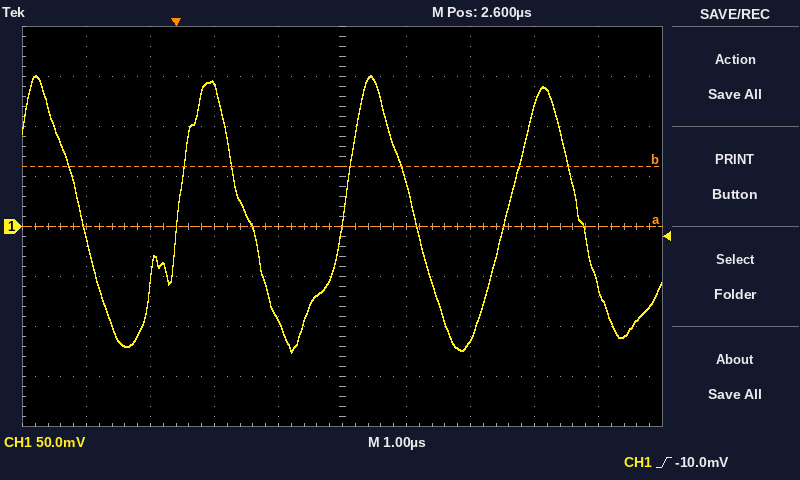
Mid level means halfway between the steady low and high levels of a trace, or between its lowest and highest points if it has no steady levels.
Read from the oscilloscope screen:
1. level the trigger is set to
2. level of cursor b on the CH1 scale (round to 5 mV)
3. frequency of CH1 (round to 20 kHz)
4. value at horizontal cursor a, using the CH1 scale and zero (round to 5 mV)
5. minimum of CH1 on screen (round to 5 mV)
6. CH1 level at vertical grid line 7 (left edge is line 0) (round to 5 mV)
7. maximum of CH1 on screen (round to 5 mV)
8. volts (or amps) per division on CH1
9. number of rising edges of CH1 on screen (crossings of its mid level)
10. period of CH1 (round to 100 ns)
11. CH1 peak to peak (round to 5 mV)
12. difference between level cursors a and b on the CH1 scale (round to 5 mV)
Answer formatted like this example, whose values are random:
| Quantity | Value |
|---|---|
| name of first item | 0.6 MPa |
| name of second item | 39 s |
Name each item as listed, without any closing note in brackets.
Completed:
| Quantity | Value |
|---|---|
| level the trigger is set to | -10.0 mV |
| level of cursor b on the CH1 scale | 60 mV |
| frequency of CH1 | 380 kHz |
| value at horizontal cursor a, using the CH1 scale and zero | 0 mV |
| minimum of CH1 on screen | -125 mV |
| CH1 level at vertical grid line 7 (left edge is line 0) | -115 mV |
| maximum of CH1 on screen | 150 mV |
| volts (or amps) per division on CH1 | 50 mV |
| number of rising edges of CH1 on screen | 3 |
| period of CH1 | 2.6 µs |
| CH1 peak to peak | 275 mV |
| difference between level cursors a and b on the CH1 scale | 60 mV |
